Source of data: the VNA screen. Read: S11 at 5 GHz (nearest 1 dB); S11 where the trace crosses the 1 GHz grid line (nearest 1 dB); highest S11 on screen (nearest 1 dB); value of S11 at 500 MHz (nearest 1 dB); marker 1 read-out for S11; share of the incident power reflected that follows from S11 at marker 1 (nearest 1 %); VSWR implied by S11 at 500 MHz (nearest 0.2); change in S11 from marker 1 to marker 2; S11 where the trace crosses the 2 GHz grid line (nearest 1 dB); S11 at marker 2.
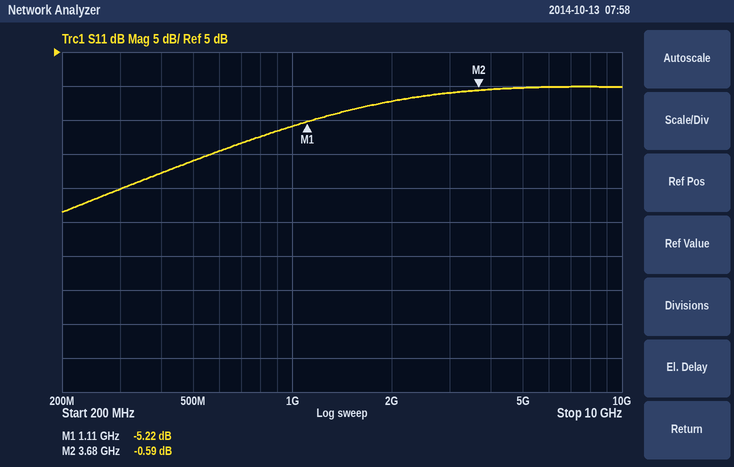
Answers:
0 dB
-6 dB
0 dB
-11 dB
-5.22 dB
30 %
1.8
4.63 dB
-2 dB
-0.59 dB
